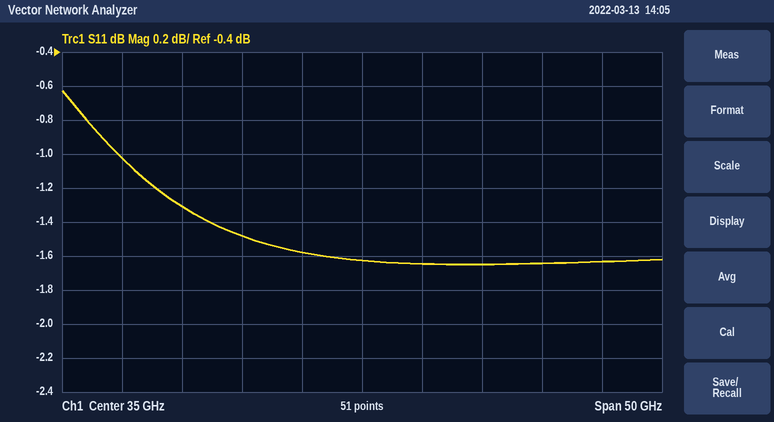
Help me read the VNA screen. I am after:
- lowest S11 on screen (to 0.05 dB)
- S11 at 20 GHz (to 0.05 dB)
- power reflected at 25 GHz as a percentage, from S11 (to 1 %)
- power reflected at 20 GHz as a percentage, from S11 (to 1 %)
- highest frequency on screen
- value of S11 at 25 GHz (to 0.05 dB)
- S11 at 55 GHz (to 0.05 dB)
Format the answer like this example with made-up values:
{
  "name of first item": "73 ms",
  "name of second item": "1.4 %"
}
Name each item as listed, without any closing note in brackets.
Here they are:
{
  "lowest S11 on screen": "-1.65 dB",
  "S11 at 20 GHz": "-1.30 dB",
  "power reflected at 25 GHz as a percentage, from S11": "71 %",
  "power reflected at 20 GHz as a percentage, from S11": "74 %",
  "highest frequency on screen": "60 GHz",
  "value of S11 at 25 GHz": "-1.50 dB",
  "S11 at 55 GHz": "-1.65 dB"
}
